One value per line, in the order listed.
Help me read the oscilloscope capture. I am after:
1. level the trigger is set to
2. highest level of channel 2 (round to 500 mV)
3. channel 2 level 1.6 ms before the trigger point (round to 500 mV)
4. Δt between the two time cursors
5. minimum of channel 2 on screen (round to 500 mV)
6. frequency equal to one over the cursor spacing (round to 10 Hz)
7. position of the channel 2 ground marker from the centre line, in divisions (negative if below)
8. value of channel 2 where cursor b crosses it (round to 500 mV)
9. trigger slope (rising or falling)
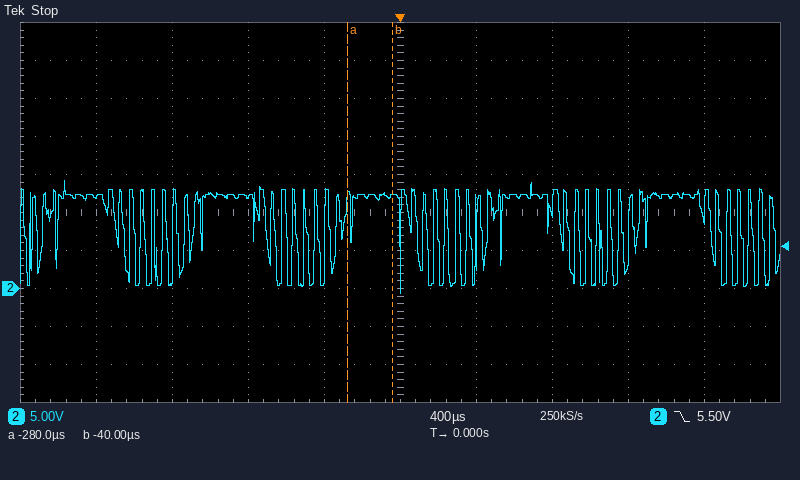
5.50 V
14.0 V
12.0 V
240 µs
-500 mV
4.17 kHz
-2.0 div
12.0 V
falling
